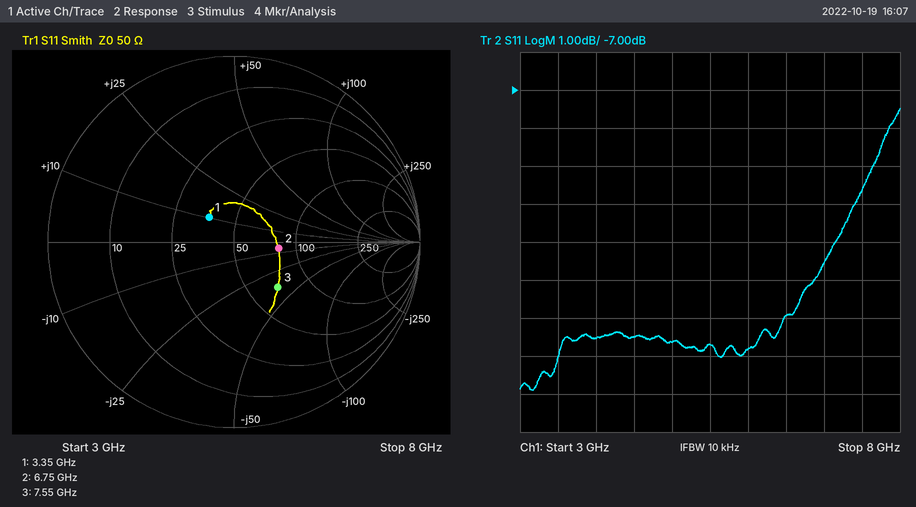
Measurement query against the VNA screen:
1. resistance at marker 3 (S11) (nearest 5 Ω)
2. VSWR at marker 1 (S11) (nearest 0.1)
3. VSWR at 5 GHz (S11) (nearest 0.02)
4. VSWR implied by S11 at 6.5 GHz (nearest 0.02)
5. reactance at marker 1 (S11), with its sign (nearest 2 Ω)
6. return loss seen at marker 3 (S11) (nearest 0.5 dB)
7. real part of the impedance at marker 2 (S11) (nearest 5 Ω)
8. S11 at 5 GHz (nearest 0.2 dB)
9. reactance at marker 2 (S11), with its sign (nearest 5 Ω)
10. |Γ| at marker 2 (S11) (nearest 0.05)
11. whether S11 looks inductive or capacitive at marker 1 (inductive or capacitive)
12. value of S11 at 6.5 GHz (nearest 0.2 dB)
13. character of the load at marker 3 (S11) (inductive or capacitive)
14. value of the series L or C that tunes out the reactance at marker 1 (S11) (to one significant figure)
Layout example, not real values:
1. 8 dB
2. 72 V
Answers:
1. 70 Ω
2. 1.5
3. 1.52
4. 1.58
5. +10 Ω
6. 9.5 dB
7. 80 Ω
8. -13.6 dB
9. -5 Ω
10. 0.25
11. inductive
12. -13.0 dB
13. capacitive
14. 5 pF
